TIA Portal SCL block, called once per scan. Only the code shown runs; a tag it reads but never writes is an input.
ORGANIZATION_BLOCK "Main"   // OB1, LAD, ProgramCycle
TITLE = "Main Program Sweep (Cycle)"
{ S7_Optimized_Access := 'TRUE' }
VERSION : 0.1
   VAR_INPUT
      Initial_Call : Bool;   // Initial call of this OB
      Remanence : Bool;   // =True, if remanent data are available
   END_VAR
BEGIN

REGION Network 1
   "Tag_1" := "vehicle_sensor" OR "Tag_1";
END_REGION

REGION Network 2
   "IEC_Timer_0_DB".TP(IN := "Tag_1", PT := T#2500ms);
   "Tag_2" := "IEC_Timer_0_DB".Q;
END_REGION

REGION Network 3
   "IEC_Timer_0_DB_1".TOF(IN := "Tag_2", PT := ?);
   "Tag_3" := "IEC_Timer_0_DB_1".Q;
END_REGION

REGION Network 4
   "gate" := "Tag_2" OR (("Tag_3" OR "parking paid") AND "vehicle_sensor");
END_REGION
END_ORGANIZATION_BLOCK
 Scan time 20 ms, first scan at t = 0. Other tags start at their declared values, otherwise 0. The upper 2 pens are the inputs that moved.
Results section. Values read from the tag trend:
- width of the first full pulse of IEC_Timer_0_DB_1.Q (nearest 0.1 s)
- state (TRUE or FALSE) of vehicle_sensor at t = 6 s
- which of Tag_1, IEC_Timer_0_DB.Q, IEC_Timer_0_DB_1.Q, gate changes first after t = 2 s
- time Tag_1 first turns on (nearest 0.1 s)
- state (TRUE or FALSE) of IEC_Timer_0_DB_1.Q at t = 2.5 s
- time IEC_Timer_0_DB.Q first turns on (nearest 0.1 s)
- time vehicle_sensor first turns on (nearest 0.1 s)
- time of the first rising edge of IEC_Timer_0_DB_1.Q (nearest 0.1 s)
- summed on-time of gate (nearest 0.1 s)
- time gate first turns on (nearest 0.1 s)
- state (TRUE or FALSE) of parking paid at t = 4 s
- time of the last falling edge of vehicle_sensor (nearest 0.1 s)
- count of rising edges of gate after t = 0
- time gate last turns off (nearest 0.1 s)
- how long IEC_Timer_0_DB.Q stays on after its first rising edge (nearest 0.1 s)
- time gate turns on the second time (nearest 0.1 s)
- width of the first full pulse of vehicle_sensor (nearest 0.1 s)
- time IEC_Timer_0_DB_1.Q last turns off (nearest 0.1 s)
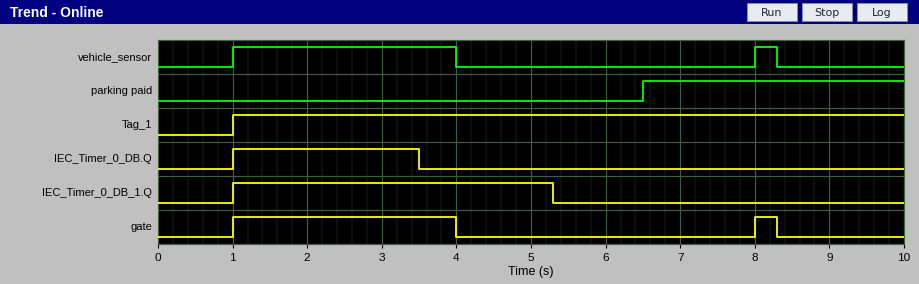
4.3 s
FALSE
IEC_Timer_0_DB.Q
1.0 s
TRUE
1.0 s
1.0 s
1.0 s
3.3 s
1.0 s
FALSE
8.3 s
2
8.3 s
2.5 s
8.0 s
3.0 s
5.3 s
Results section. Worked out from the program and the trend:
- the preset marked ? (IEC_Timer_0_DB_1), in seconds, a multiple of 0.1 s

1.8 s
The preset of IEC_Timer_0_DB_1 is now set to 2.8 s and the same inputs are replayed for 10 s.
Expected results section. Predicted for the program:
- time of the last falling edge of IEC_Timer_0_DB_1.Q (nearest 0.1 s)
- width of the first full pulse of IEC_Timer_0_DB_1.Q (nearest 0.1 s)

6.3 s
5.3 s
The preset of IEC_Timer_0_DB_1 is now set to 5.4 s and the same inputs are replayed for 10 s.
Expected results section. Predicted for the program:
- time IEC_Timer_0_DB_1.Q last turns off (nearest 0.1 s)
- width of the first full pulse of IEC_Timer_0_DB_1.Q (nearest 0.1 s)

8.9 s
7.9 s
